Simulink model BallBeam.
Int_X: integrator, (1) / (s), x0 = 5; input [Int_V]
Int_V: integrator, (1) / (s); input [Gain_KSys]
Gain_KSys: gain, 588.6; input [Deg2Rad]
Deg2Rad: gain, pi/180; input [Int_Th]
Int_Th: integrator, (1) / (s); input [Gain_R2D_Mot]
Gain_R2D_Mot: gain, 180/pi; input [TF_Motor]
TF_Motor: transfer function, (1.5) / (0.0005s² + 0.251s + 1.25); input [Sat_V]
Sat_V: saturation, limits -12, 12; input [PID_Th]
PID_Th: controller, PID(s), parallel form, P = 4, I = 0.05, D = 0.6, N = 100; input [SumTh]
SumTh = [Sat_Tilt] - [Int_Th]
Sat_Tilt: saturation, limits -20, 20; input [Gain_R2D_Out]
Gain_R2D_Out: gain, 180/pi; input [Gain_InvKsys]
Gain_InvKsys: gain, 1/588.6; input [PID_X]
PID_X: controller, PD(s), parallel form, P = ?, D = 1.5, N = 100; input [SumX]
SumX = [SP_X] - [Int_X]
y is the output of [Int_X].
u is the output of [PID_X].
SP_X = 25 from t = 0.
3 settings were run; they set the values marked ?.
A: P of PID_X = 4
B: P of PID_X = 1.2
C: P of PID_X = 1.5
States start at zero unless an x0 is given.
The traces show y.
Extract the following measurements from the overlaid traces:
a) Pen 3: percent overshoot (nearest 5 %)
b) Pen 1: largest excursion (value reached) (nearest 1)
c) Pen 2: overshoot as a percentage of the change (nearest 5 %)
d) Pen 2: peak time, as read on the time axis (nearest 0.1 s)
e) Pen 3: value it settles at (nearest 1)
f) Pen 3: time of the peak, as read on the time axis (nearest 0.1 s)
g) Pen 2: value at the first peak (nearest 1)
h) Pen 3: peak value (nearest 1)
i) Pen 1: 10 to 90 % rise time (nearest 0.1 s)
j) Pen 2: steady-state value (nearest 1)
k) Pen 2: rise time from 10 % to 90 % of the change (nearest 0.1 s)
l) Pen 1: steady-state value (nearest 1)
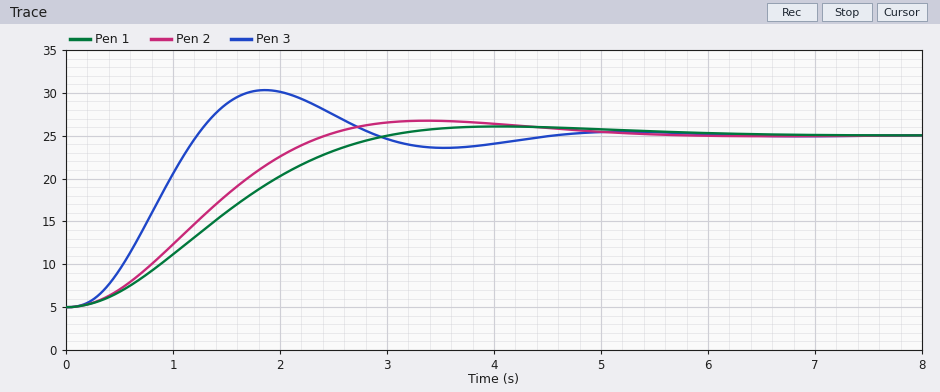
25 %
26
10 %
3.4 s
25
1.9 s
27
30
1.9 s
25
1.6 s
25
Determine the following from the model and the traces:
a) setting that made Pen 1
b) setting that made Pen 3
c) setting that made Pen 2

B
A
C
